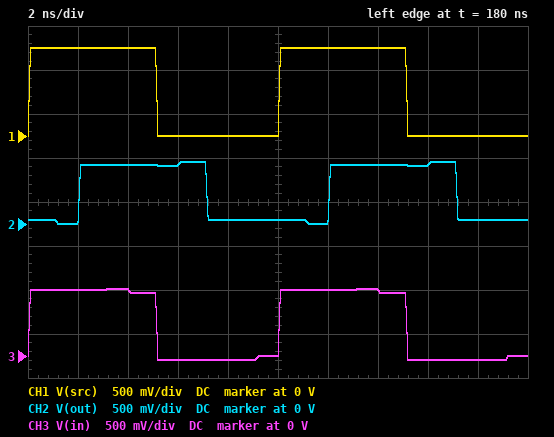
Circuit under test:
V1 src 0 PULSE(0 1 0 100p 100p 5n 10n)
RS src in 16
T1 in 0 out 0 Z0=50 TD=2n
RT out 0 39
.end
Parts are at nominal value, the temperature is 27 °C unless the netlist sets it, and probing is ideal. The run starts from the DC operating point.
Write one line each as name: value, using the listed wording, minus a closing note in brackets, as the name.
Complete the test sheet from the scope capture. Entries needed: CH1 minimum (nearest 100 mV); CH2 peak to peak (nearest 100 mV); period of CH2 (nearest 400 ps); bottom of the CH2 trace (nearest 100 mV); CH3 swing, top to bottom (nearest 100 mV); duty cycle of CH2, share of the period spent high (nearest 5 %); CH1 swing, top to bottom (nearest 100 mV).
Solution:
CH1 minimum: 0 V
CH2 peak to peak: 700 mV
period of CH2: 10.0 ns
bottom of the CH2 trace: 0 V
CH3 swing, top to bottom: 800 mV
duty cycle of CH2, share of the period spent high: 50 %
CH1 swing, top to bottom: 1.0 V
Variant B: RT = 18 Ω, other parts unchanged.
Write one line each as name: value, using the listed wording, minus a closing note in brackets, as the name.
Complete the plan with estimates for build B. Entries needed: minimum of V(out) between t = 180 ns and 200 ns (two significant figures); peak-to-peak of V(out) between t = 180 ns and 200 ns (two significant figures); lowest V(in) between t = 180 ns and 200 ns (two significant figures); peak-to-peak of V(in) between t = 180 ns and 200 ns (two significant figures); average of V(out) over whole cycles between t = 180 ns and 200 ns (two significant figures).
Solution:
minimum of V(out) between t = 180 ns and 200 ns: 25 mV
peak-to-peak of V(out) between t = 180 ns and 200 ns: 480 mV
lowest V(in) between t = 180 ns and 200 ns: -220 mV
peak-to-peak of V(in) between t = 180 ns and 200 ns: 960 mV
average of V(out) over whole cycles between t = 180 ns and 200 ns: 270 mV
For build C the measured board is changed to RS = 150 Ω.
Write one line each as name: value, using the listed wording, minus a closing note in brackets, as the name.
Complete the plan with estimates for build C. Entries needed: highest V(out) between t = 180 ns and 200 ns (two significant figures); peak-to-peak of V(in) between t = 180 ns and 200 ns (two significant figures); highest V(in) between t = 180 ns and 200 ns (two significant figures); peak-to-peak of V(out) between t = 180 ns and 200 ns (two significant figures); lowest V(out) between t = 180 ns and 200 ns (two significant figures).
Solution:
highest V(out) between t = 180 ns and 200 ns: 220 mV
peak-to-peak of V(in) between t = 180 ns and 200 ns: 300 mV
highest V(in) between t = 180 ns and 200 ns: 250 mV
peak-to-peak of V(out) between t = 180 ns and 200 ns: 230 mV
lowest V(out) between t = 180 ns and 200 ns: -14 mV
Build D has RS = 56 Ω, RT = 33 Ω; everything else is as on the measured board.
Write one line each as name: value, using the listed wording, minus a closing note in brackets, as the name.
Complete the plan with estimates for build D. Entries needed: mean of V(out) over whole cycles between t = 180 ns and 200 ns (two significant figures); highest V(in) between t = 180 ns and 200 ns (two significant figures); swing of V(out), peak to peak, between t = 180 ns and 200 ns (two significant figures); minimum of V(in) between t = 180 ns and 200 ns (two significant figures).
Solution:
mean of V(out) over whole cycles between t = 180 ns and 200 ns: 190 mV
highest V(in) between t = 180 ns and 200 ns: 470 mV
swing of V(out), peak to peak, between t = 180 ns and 200 ns: 380 mV
minimum of V(in) between t = 180 ns and 200 ns: -100 mV
